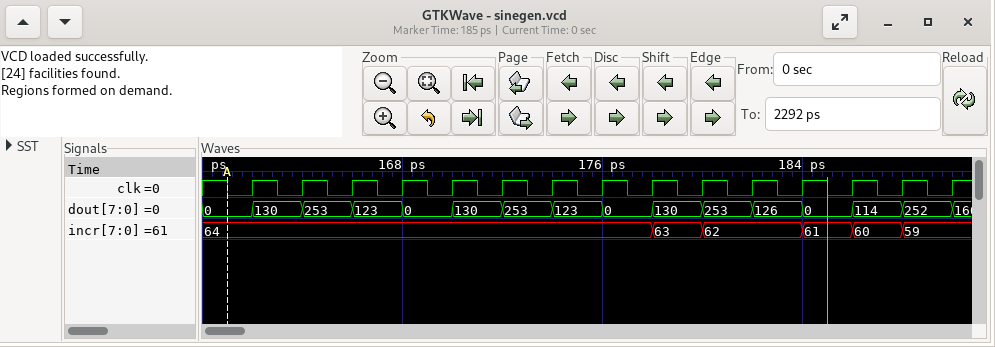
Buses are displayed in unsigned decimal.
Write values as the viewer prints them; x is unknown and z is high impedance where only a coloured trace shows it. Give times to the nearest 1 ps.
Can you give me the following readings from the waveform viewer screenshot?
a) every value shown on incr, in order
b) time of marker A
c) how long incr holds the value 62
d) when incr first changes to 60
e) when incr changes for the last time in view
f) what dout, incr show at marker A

64, 63, 62, 61, 60, 59
161 ps
4 ps
186 ps
188 ps
dout=0, incr=64
